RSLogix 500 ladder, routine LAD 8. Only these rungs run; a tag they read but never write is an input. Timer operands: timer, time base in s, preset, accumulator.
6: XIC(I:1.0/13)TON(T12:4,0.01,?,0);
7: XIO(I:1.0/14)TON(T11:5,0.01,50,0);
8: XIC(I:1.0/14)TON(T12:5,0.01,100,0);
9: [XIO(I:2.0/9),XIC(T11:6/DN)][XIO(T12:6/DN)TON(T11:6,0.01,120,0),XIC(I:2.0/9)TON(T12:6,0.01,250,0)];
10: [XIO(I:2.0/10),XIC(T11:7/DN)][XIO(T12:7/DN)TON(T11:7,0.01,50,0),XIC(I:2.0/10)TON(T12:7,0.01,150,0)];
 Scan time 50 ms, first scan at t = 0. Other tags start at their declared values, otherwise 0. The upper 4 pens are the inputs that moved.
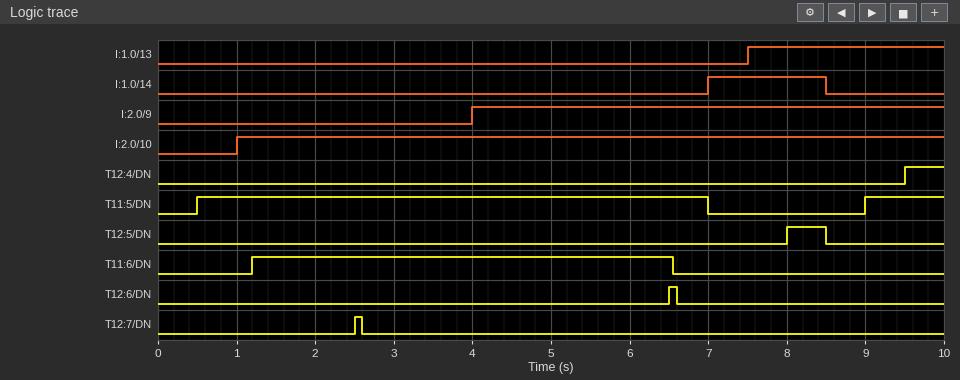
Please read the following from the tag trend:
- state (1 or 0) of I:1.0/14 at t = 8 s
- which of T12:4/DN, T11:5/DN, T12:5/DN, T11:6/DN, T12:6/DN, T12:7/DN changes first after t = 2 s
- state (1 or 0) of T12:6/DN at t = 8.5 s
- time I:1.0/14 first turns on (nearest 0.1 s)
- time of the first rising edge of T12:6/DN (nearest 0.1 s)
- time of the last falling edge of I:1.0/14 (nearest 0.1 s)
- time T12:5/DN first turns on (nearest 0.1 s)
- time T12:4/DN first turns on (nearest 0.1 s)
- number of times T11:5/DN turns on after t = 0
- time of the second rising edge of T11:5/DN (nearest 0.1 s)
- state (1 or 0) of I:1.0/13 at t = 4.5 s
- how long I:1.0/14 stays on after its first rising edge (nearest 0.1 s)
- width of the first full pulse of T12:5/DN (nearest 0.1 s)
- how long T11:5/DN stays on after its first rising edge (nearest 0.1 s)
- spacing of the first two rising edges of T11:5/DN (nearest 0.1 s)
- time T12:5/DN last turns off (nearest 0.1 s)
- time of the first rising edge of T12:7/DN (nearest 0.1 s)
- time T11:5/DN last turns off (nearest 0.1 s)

1
T12:7/DN
0
7.0 s
6.5 s
8.5 s
8.0 s
9.5 s
2
9.0 s
0
1.5 s
0.5 s
6.5 s
8.5 s
8.5 s
2.5 s
7.0 s
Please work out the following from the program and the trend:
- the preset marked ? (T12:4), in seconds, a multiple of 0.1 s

2.0 s
